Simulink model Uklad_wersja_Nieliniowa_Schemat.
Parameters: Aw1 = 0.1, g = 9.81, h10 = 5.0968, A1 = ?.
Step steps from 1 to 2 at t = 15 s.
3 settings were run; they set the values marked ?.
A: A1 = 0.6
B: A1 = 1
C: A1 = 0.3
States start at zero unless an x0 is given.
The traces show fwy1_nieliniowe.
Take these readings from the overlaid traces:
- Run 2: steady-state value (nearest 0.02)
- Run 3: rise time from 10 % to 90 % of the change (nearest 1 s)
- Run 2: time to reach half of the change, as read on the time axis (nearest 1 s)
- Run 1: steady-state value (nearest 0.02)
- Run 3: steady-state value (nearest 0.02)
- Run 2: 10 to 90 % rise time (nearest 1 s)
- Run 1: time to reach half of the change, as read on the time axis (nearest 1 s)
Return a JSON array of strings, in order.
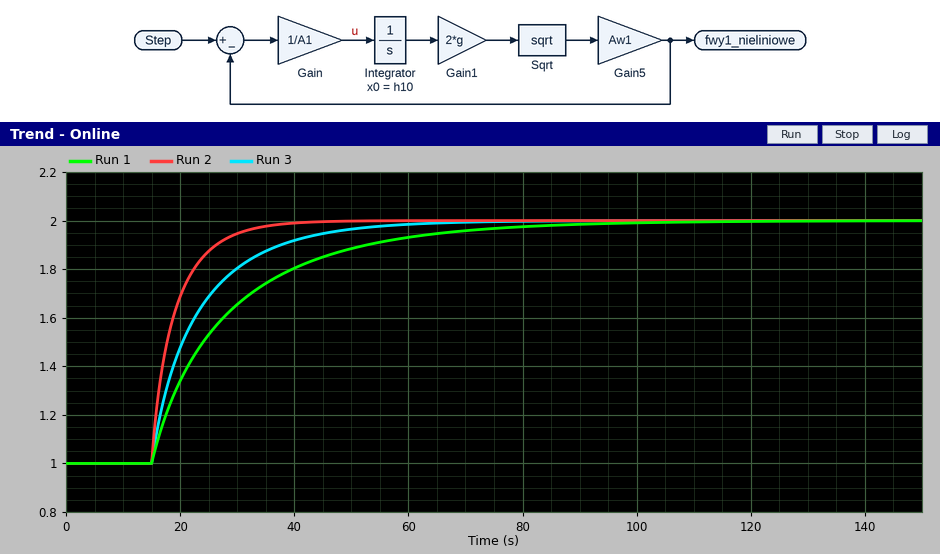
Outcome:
["2.00", "22 s", "18 s", "2.00", "2.00", "11 s", "24 s"]
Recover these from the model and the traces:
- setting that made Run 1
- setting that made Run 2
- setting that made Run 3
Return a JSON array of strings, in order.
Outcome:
["B", "C", "A"]
